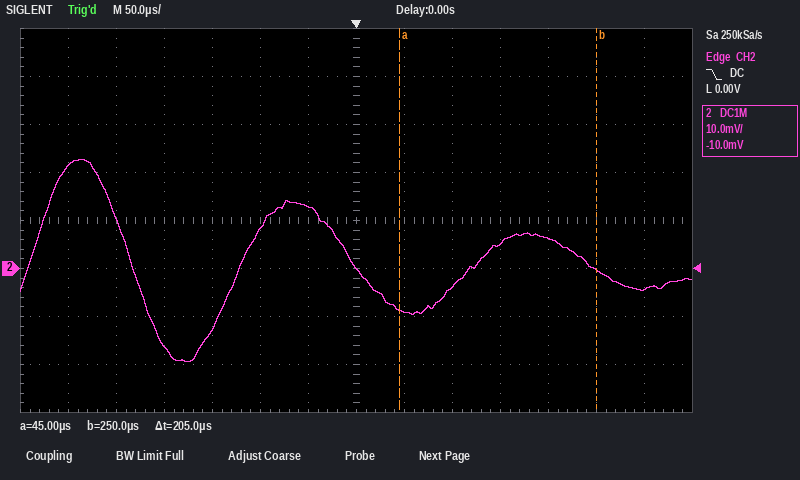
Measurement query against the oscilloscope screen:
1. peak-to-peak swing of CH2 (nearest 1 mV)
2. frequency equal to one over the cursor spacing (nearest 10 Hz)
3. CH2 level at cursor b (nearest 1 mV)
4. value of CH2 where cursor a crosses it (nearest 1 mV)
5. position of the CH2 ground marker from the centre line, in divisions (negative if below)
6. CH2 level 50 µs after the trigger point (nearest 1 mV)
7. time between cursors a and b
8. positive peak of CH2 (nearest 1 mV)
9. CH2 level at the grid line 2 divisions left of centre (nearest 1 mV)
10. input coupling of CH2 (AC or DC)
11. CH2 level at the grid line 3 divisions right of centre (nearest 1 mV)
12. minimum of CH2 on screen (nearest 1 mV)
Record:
42 mV
4.88 kHz
0 mV
-9 mV
-1.0 div
-9 mV
205 µs
23 mV
8 mV
DC
5 mV
-19 mV
